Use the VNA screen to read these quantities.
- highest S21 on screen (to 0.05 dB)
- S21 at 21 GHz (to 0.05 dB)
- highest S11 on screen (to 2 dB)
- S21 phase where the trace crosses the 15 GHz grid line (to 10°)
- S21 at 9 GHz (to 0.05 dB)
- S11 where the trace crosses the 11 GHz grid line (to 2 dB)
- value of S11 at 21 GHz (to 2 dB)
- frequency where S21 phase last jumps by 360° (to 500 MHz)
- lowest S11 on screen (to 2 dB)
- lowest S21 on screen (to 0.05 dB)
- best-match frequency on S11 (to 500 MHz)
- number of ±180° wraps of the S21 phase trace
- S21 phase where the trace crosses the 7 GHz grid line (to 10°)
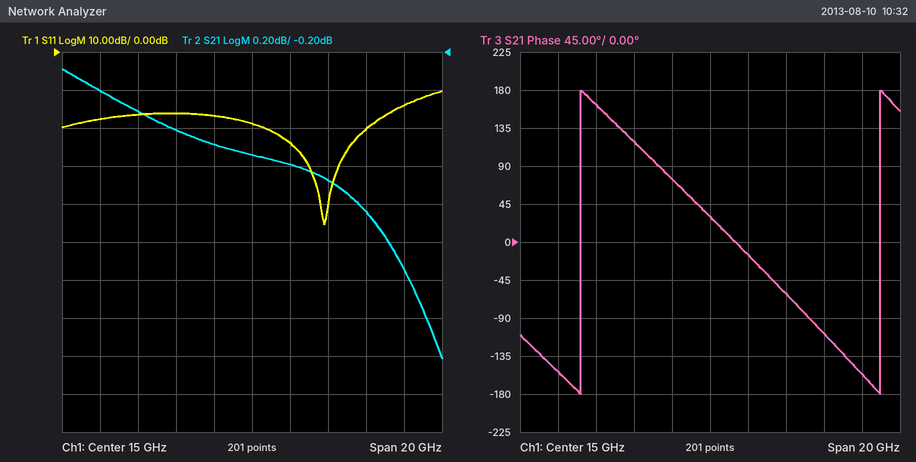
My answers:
-0.30 dB
-1.05 dB
-10 dB
30°
-0.50 dB
-16 dB
-20 dB
24.0 GHz
-46 dB
-1.80 dB
19.0 GHz
2
-150°
